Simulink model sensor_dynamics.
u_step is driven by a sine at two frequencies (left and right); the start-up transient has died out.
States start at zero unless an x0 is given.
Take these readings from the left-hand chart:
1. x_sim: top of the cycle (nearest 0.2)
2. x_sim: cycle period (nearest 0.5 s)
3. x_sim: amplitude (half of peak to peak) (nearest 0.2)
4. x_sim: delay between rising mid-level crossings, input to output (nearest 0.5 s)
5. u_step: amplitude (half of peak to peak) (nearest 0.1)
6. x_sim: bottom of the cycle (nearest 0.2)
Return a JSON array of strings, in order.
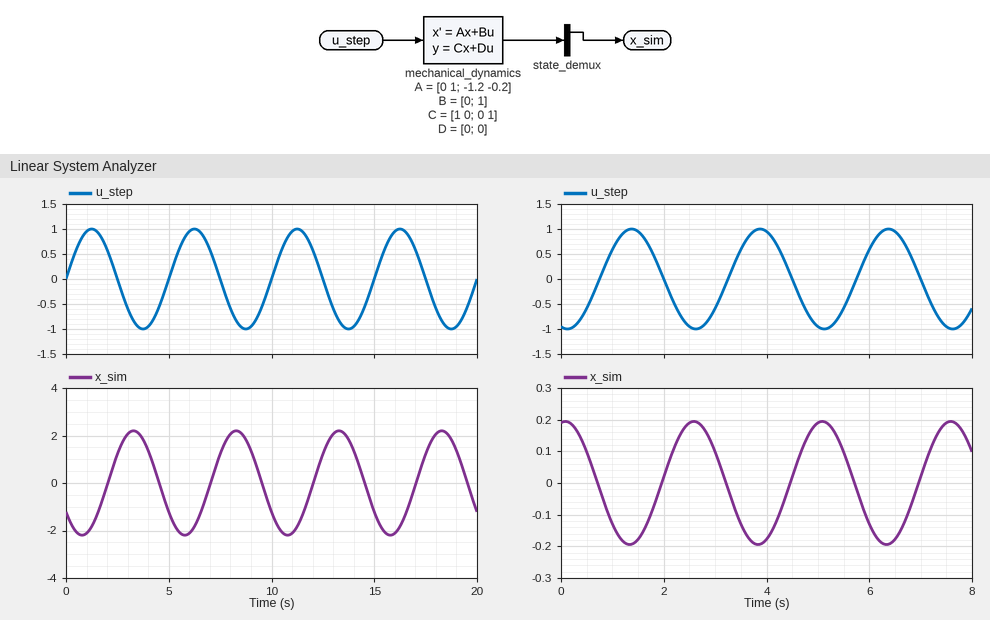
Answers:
["2.2", "5.0 s", "2.2", "2.0 s", "1.0", "-2.2"]
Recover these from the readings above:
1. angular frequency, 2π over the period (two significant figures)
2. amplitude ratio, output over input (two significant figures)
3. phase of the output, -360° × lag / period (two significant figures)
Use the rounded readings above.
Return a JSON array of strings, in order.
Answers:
["1.3 rad/s", "2.2", "-140°"]
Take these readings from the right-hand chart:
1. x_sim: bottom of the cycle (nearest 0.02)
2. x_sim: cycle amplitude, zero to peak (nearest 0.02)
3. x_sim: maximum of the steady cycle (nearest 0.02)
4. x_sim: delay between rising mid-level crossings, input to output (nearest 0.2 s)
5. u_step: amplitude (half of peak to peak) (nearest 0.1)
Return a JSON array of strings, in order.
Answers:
["-0.20", "0.20", "0.20", "1.2 s", "1.0"]
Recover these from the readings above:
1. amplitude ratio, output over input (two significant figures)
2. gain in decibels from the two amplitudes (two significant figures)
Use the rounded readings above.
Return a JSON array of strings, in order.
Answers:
["0.20", "-14 dB"]
